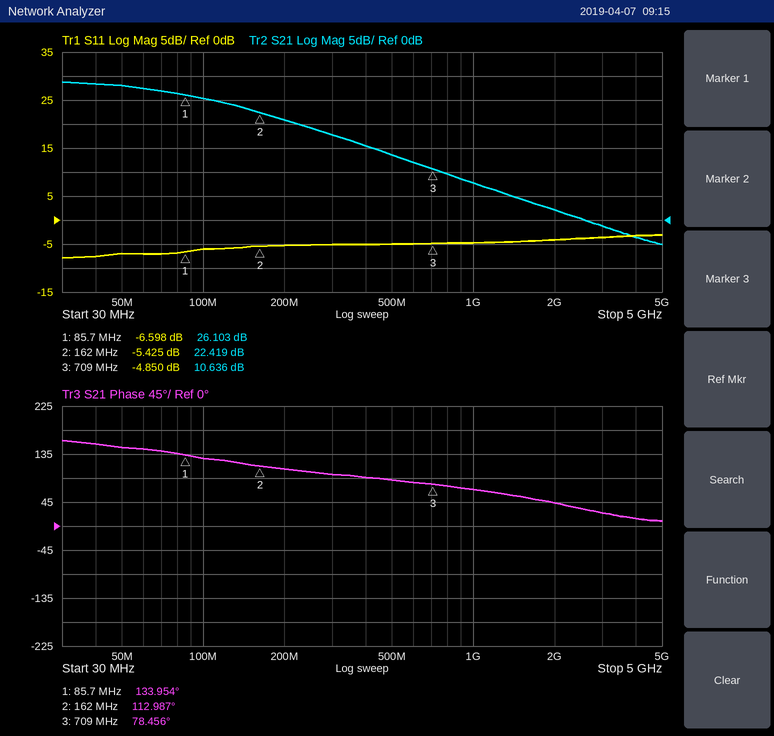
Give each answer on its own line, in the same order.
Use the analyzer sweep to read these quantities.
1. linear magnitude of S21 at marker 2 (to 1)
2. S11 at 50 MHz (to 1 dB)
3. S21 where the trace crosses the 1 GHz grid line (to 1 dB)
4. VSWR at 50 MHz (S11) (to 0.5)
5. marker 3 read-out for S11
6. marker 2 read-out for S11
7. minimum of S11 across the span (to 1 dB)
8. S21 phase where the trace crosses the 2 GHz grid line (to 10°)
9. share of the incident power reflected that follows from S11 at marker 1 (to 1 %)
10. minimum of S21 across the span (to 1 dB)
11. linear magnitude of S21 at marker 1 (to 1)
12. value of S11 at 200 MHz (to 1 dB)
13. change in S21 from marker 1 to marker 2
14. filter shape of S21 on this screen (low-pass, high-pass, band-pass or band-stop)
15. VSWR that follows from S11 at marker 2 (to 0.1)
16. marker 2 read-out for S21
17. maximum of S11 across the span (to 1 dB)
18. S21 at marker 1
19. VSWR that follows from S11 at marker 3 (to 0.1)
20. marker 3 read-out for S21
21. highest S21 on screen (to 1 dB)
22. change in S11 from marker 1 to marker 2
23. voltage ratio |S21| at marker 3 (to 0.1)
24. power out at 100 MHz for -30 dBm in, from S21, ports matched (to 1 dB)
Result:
13
-7 dB
8 dB
2.5
-4.850 dB
-5.425 dB
-8 dB
40°
22 %
-5 dB
20
-5 dB
-3.684 dB
low-pass
3.3
22.419 dB
-3 dB
26.103 dB
3.7
10.636 dB
29 dB
1.173 dB
3.4
-5 dBm
